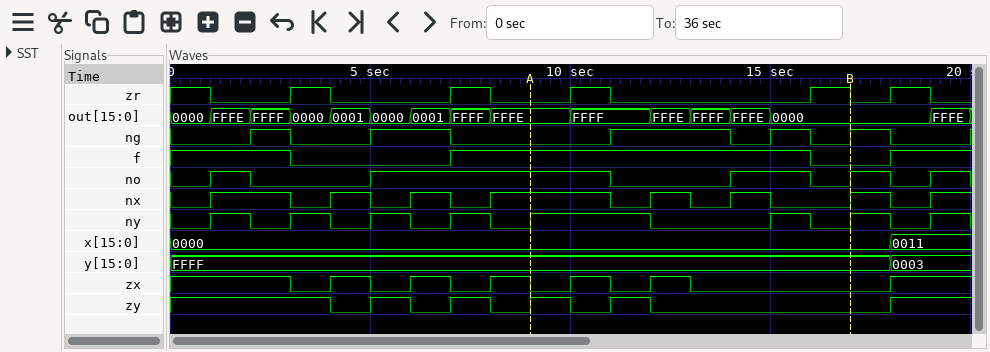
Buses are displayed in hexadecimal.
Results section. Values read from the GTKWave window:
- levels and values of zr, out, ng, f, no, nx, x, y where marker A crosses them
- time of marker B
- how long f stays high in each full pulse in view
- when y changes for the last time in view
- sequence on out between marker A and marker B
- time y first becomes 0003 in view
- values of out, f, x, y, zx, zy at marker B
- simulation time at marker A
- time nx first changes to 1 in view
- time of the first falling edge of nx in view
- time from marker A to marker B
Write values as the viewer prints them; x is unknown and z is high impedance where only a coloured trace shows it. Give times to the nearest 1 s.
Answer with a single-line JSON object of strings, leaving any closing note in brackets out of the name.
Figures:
{"levels and values of zr, out, ng, f, no, nx, x, y where marker A crosses them": "zr=0, out=FFFE, ng=0, f=1, no=1, nx=1, x=0000, y=FFFF", "time of marker B": "17 s", "how long f stays high in each full pulse in view": "9 s", "when y changes for the last time in view": "18 s", "sequence on out between marker A and marker B": "FFFE, FFFF, FFFE, FFFF, FFFE, 0000", "time y first becomes 0003 in view": "18 s", "values of out, f, x, y, zx, zy at marker B": "out=0000, f=0, x=0000, y=FFFF, zx=0, zy=0", "simulation time at marker A": "9 s", "time nx first changes to 1 in view": "1 s", "time of the first falling edge of nx in view": "3 s", "time from marker A to marker B": "8 s"}
